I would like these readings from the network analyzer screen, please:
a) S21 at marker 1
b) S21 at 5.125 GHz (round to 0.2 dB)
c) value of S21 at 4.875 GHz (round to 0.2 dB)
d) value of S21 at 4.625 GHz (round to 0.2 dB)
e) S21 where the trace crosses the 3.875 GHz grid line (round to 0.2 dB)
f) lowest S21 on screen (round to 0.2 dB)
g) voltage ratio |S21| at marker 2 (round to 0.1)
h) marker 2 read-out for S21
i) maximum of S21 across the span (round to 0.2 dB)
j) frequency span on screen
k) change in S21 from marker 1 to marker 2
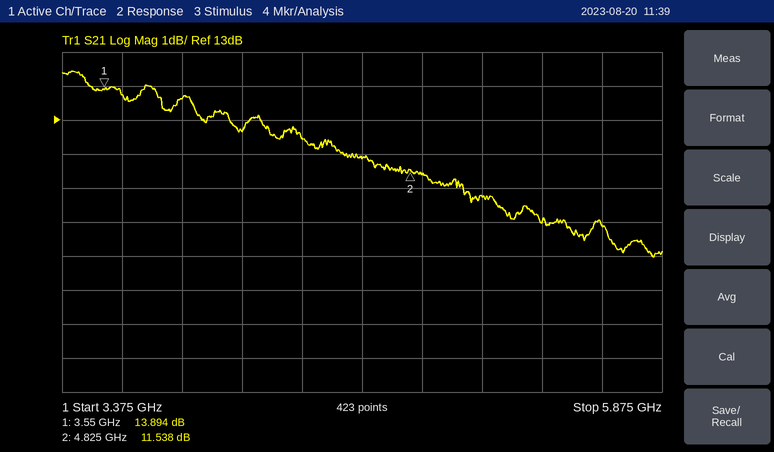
13.894 dB
10.8 dB
11.4 dB
11.8 dB
13.6 dB
9.0 dB
3.8
11.538 dB
14.4 dB
2.5 GHz
-2.356 dB
